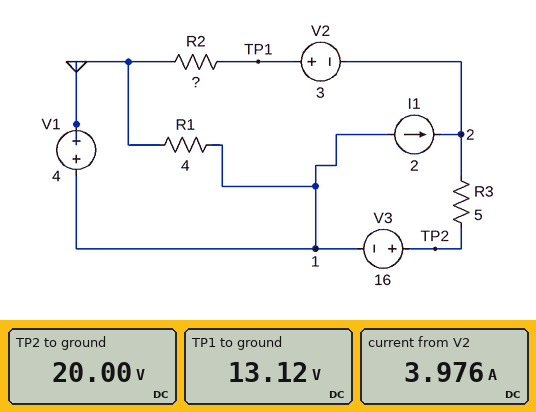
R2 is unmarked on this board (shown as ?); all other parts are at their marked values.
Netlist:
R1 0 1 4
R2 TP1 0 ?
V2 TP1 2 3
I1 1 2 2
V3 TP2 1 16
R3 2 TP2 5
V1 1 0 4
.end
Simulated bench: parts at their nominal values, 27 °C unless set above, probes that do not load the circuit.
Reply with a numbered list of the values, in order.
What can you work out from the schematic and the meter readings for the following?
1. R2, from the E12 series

1. 3.3 Ω
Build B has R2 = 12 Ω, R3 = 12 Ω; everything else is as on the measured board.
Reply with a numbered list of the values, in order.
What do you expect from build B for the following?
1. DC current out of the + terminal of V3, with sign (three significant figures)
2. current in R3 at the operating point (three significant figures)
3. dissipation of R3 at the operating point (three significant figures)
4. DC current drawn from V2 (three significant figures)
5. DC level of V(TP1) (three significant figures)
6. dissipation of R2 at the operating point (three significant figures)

1. -41.7 mA
2. 41.7 mA
3. 20.8 mW
4. 1.96 A
5. 23.5 V
6. 46.0 W
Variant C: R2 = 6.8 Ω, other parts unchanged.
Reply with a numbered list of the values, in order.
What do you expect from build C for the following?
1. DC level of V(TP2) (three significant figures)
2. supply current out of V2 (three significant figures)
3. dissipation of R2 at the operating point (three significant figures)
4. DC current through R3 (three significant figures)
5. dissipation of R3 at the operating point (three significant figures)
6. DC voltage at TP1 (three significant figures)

1. 20.0 V
2. 2.80 A
3. 53.2 W
4. 797 mA
5. 3.17 W
6. 19.0 V
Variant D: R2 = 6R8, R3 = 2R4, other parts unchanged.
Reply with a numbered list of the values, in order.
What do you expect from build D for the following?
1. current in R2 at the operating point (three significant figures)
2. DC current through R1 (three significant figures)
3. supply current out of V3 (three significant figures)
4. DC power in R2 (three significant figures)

1. 3.02 A
2. 1.00 A
3. 1.02 A
4. 62.1 W
